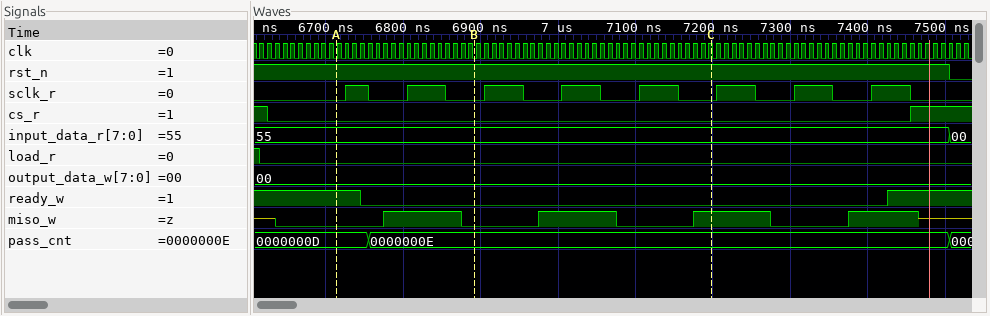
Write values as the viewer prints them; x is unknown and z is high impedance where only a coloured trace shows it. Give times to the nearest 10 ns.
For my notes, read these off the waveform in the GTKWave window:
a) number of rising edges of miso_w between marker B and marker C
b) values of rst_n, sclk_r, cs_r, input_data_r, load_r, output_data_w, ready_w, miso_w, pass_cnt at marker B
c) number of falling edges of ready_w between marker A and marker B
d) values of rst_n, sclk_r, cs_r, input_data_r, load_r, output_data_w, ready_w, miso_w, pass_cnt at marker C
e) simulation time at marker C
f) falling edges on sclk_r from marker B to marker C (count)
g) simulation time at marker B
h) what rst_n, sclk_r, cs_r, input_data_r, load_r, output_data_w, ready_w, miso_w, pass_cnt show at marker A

2
rst_n=1, sclk_r=0, cs_r=0, input_data_r=55, load_r=0, output_data_w=00, ready_w=0, miso_w=0, pass_cnt=0000000E
1
rst_n=1, sclk_r=0, cs_r=0, input_data_r=55, load_r=0, output_data_w=00, ready_w=0, miso_w=1, pass_cnt=0000000E
7200 ns
3
6890 ns
rst_n=1, sclk_r=0, cs_r=0, input_data_r=55, load_r=0, output_data_w=00, ready_w=1, miso_w=0, pass_cnt=0000000D
